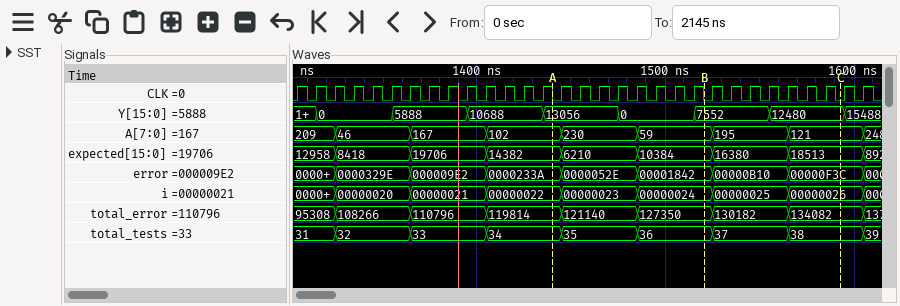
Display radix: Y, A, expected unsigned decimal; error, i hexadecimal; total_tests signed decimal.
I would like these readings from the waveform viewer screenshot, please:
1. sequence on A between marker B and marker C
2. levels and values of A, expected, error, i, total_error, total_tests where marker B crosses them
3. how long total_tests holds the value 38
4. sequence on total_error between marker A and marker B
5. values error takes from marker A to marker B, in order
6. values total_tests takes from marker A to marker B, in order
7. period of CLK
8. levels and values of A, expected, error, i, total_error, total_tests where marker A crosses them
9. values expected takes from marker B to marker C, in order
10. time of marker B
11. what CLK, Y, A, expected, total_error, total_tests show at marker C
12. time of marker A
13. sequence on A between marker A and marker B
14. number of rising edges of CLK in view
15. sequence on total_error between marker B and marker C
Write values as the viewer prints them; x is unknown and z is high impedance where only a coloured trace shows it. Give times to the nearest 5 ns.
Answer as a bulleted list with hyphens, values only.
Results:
- 59, 195, 121
- A=59, expected=10384, error=00001842, i=00000024, total_error=127350, total_tests=36
- 40 ns
- 119814, 121140, 127350
- 0000233A, 0000052E, 00001842
- 34, 35, 36
- 10 ns
- A=102, expected=14382, error=0000233A, i=00000022, total_error=119814, total_tests=34
- 10384, 16380, 18513
- 1520 ns
- CLK=0, Y=12480, A=121, expected=18513, total_error=134082, total_tests=38
- 1440 ns
- 102, 230, 59
- 31
- 127350, 130182, 134082
